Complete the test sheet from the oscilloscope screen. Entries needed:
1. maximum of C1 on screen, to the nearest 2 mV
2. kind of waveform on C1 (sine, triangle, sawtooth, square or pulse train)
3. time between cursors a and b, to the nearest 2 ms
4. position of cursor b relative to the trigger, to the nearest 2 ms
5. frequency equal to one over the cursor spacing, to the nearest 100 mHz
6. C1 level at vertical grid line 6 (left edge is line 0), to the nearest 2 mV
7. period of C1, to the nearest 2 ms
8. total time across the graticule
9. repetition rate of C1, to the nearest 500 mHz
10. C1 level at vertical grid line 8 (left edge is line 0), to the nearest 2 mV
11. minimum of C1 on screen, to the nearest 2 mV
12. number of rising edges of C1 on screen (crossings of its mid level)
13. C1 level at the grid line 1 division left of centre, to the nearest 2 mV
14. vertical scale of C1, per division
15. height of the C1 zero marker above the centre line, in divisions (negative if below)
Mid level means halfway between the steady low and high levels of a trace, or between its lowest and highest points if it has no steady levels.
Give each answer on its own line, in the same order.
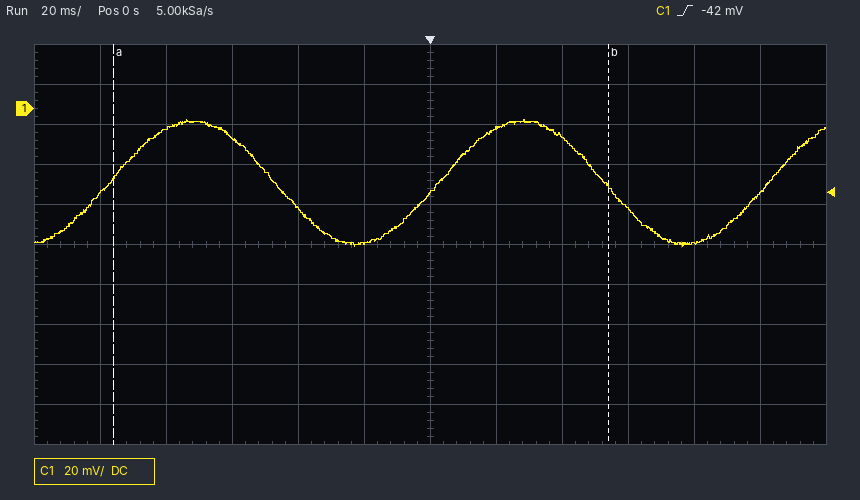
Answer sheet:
-6 mV
sine
150 ms
+54 ms
6.7 Hz
-42 mV
100 ms
240 ms
10.0 Hz
-14 mV
-68 mV
3
-68 mV
20 mV
+3.4 div
